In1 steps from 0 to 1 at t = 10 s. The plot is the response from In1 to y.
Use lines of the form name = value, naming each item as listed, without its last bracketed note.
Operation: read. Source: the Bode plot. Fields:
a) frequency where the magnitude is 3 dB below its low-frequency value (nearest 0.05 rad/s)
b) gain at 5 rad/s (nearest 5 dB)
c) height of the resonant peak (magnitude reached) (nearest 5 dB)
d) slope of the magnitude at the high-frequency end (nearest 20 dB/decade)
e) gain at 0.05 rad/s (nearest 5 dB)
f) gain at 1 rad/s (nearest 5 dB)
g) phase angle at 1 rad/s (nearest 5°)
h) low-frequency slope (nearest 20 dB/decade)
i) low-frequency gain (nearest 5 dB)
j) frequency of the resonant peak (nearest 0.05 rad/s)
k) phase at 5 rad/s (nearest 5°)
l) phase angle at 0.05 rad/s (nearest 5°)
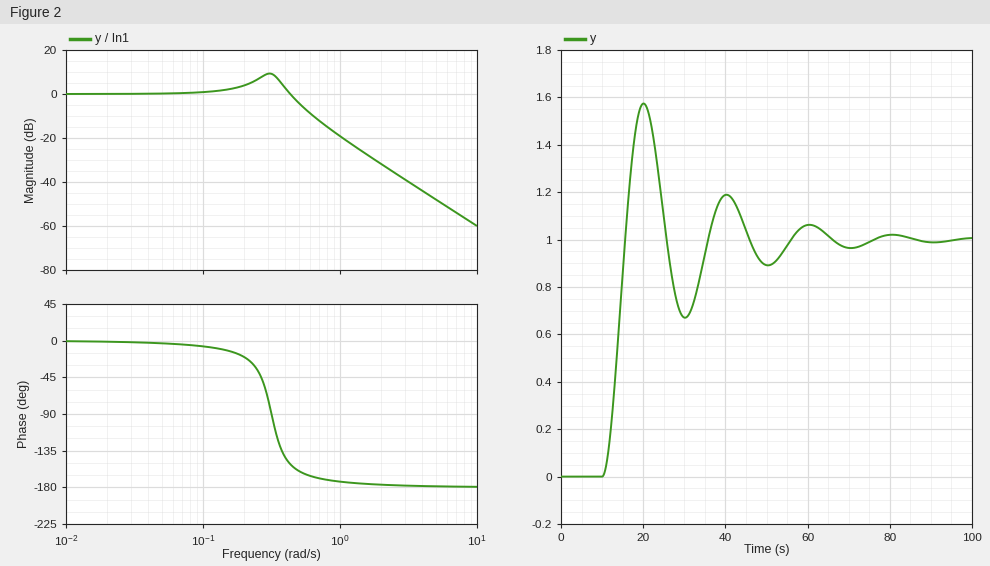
frequency where the magnitude is 3 dB below its low-frequency value = 0.50 rad/s
gain at 5 rad/s = -50 dB
height of the resonant peak (magnitude reached) = 10 dB
slope of the magnitude at the high-frequency end = -40 dB/decade
gain at 0.05 rad/s = 0 dB
gain at 1 rad/s = -20 dB
phase angle at 1 rad/s = -175°
low-frequency slope = 0 dB/decade
low-frequency gain = 0 dB
frequency of the resonant peak = 0.30 rad/s
phase at 5 rad/s = -180°
phase angle at 0.05 rad/s = -5°
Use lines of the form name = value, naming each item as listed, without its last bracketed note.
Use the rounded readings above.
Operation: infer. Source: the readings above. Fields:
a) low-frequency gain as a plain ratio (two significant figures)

low-frequency gain as a plain ratio = 1.0
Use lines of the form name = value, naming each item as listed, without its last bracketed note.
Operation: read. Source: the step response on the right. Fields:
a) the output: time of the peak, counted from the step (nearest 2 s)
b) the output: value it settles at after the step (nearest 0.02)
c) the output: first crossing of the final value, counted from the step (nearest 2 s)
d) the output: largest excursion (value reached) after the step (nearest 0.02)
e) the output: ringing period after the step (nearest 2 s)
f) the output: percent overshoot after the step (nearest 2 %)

the output: time of the peak, counted from the step = 10 s
the output: value it settles at after the step = 1.00
the output: first crossing of the final value, counted from the step = 6 s
the output: largest excursion (value reached) after the step = 1.58
the output: ringing period after the step = 20 s
the output: percent overshoot after the step = 58 %
